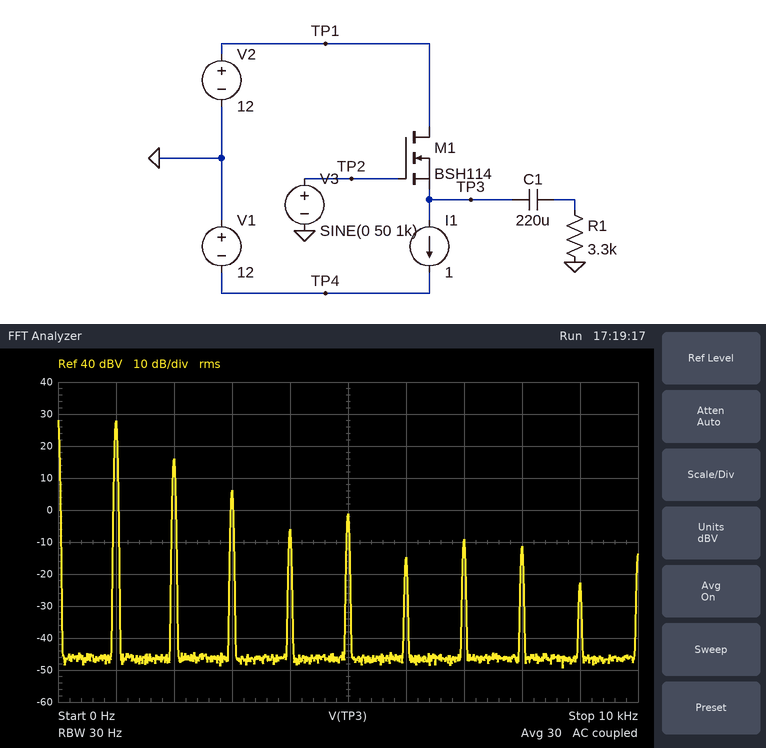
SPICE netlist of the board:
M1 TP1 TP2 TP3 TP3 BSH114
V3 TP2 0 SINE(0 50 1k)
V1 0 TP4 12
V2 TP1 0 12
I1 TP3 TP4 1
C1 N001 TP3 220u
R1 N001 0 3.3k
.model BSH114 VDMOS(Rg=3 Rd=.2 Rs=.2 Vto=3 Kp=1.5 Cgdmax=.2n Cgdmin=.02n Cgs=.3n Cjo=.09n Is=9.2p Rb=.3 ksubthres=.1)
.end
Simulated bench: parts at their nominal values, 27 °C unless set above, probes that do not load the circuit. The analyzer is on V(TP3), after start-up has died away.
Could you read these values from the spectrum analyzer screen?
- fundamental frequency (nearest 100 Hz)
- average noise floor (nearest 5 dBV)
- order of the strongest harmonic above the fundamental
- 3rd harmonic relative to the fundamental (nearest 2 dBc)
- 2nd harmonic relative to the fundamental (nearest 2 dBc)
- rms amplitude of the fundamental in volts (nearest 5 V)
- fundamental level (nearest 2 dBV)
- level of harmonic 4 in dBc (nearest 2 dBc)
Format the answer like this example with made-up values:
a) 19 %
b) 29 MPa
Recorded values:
a) 1.0 kHz
b) -45 dBV
c) 2
d) -22 dBc
e) -12 dBc
f) 25 V
g) 28 dBV
h) -34 dBc
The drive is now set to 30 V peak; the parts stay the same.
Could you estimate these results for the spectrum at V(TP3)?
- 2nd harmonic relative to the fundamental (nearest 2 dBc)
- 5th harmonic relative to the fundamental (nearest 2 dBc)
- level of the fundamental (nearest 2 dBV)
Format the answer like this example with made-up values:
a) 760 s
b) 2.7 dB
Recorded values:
a) -16 dBc
b) -38 dBc
c) 24 dBV
